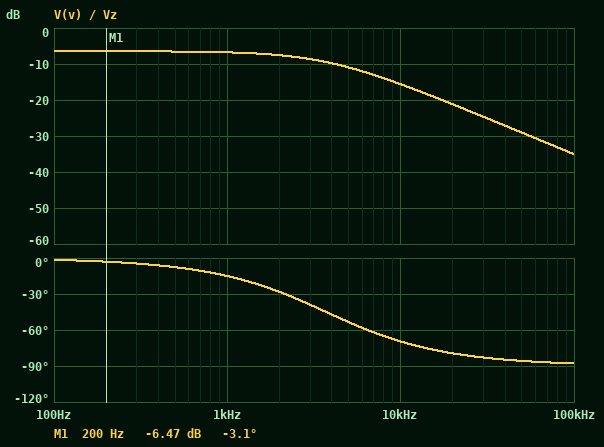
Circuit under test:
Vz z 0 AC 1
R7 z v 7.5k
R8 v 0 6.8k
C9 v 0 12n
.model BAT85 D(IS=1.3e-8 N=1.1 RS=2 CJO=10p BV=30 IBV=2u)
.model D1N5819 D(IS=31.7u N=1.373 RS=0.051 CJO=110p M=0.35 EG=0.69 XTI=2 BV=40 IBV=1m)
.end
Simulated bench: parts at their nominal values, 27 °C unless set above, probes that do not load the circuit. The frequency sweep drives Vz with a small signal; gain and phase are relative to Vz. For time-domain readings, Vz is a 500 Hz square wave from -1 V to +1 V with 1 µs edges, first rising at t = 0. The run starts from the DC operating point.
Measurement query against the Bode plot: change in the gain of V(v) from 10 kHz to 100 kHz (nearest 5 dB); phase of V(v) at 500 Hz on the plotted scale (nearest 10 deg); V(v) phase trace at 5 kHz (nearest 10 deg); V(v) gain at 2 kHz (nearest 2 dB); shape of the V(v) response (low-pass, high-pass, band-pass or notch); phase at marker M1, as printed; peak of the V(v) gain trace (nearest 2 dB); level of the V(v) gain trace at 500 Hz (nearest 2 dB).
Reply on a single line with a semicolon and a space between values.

-20 dB; -10 deg; -50 deg; -8 dB; low-pass; -3.1 deg; -6 dB; -6 dB
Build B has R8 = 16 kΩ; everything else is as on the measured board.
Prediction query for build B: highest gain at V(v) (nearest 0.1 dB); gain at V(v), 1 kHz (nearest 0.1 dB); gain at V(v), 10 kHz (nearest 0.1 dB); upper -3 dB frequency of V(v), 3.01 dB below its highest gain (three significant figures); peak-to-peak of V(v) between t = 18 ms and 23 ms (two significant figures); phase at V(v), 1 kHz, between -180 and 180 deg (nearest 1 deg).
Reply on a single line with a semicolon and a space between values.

-3.3 dB; -3.9 dB; -15.3 dB; 2.60 kHz; 1.4 V; -21 deg
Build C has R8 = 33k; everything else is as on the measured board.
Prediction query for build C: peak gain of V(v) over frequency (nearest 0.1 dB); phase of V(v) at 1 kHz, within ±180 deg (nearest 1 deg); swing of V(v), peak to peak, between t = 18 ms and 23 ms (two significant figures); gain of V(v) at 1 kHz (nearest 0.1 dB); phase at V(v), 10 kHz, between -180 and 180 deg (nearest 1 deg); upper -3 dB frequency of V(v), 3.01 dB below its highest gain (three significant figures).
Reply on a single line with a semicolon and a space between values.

-1.8 dB; -25 deg; 1.6 V; -2.6 dB; -78 deg; 2.17 kHz
